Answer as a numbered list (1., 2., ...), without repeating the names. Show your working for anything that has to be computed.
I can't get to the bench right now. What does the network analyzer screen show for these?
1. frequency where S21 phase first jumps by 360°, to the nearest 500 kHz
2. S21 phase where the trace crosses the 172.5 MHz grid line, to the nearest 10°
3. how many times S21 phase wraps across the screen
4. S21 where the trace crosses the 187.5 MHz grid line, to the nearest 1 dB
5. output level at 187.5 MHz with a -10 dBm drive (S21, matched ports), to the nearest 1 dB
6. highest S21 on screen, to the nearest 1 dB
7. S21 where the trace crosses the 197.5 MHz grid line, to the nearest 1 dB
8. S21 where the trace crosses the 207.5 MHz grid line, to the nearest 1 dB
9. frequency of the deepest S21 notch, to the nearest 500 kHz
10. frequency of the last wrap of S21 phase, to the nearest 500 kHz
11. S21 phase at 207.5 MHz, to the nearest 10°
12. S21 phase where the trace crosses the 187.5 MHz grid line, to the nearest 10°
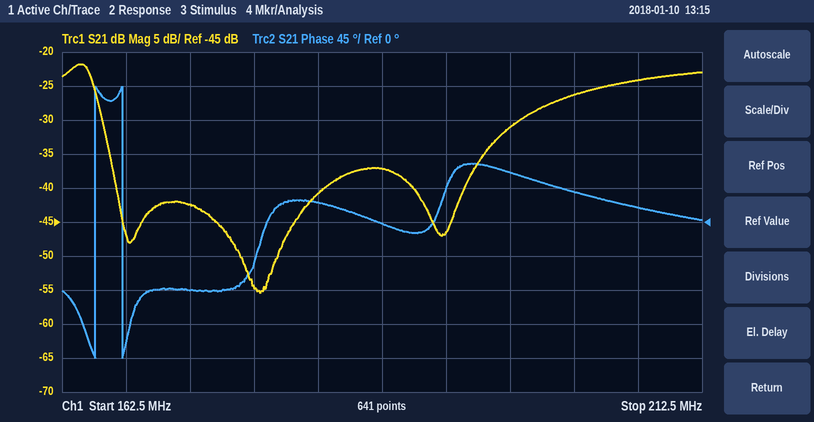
1. 165.0 MHz
2. -90°
3. 2
4. -37 dB
5. -10 dBm + (-37 dB) = -47 dBm
6. -22 dB
7. -31 dB
8. -24 dB
9. 178.0 MHz
10. 167.0 MHz
11. 20°
12. 0°
